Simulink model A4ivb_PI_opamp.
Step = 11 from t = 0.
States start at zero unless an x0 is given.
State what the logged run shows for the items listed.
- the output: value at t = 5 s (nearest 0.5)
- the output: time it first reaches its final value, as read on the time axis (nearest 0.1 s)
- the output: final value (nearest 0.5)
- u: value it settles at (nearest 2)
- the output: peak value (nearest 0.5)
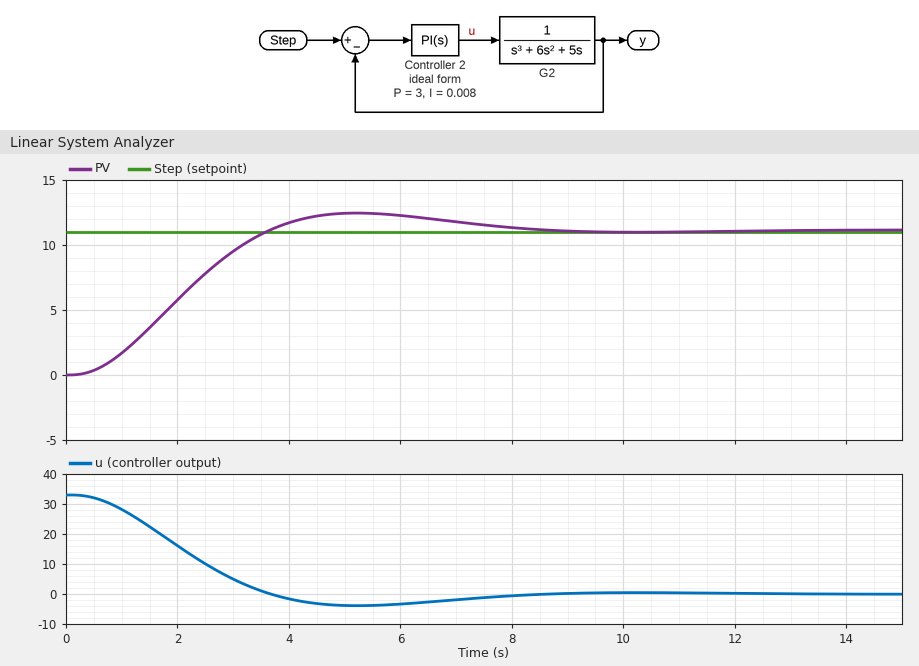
12.5
3.6 s
11.0
0
12.5
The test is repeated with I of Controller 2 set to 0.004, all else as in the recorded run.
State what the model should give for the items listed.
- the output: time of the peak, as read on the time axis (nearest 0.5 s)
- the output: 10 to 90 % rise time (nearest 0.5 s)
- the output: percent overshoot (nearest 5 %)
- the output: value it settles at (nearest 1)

5.0 s
2.5 s
10 %
11
